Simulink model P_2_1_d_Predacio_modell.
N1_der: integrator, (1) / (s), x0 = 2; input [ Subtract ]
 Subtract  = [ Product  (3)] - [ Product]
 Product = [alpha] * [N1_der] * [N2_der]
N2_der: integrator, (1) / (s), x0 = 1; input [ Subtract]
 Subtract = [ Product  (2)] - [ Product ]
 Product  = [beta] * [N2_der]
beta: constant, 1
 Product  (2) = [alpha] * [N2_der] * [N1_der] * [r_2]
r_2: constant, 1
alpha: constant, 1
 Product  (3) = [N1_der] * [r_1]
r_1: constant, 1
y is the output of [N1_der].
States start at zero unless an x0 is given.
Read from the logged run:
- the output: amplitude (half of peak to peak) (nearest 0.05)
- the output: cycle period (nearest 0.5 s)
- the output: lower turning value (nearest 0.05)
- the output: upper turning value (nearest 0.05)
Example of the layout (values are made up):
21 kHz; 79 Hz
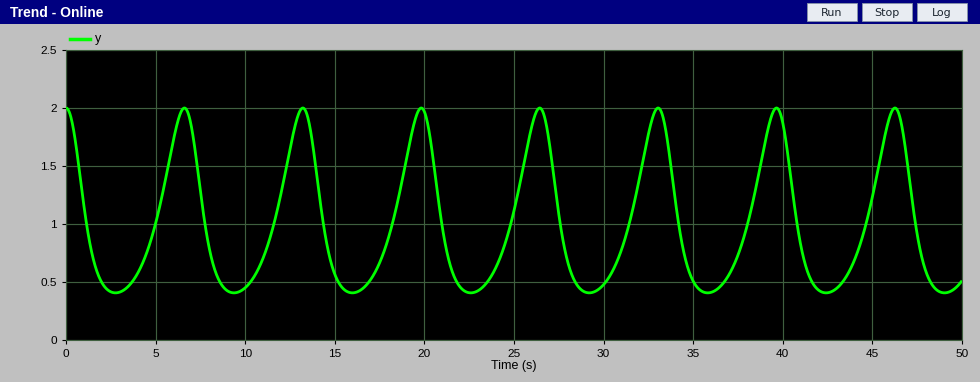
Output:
0.80; 6.5 s; 0.40; 2.00
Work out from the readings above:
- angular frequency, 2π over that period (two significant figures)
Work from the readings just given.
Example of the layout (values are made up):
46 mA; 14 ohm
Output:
0.97 rad/s
